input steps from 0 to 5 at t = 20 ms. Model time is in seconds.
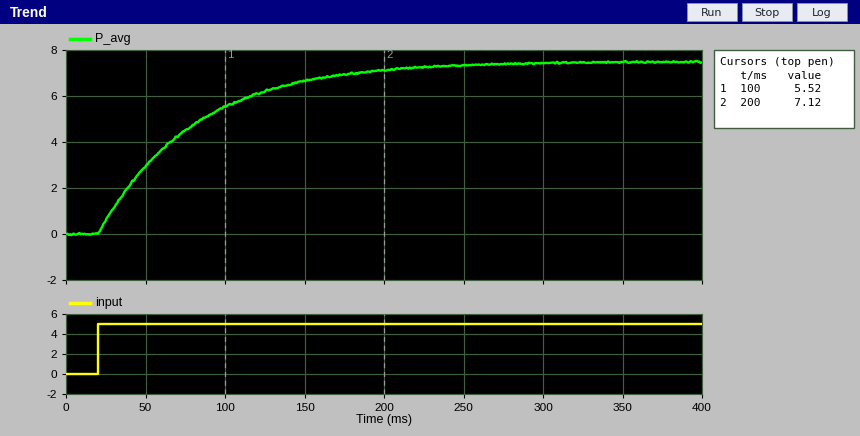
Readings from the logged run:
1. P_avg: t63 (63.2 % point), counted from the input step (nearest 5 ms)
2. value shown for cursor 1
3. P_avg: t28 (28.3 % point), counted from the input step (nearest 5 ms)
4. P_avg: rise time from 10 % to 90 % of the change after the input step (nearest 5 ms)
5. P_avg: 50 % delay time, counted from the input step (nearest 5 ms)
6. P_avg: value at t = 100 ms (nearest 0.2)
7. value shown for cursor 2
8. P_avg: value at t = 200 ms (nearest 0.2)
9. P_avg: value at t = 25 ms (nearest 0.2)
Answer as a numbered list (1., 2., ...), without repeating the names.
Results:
1. 60 ms
2. 5.52
3. 20 ms
4. 130 ms
5. 40 ms
6. 5.6
7. 7.12
8. 7.2
9. 0.6
